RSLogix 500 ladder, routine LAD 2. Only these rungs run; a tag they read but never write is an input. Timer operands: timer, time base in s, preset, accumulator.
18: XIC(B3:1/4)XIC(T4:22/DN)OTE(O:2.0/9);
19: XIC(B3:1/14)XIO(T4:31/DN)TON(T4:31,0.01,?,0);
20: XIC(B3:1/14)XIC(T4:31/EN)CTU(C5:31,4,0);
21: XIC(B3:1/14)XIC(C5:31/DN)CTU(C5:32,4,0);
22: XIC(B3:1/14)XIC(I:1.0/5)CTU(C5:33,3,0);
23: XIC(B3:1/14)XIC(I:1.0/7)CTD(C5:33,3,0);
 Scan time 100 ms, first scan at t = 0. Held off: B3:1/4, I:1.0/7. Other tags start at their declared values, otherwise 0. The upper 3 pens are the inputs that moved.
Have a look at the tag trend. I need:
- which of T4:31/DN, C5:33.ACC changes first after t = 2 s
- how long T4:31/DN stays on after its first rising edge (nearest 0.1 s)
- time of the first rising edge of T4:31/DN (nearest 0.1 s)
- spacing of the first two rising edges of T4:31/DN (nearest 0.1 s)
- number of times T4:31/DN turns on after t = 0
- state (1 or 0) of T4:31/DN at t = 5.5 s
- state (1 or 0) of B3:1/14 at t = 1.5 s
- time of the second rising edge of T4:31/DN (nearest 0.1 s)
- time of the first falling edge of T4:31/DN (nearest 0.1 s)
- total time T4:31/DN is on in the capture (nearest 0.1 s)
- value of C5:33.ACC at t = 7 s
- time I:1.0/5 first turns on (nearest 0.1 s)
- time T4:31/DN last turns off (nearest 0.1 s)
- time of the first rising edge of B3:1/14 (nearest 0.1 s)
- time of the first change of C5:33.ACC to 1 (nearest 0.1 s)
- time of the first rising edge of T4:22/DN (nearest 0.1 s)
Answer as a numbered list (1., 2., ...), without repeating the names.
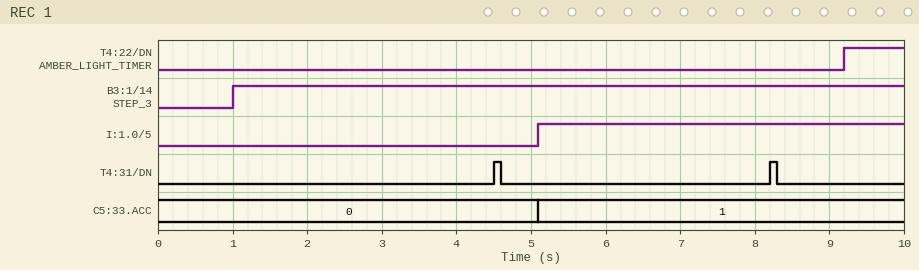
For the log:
1. T4:31/DN
2. 0.1 s
3. 4.5 s
4. 3.7 s
5. 2
6. 0
7. 1
8. 8.2 s
9. 4.6 s
10. 0.2 s
11. 1
12. 5.1 s
13. 8.3 s
14. 1.0 s
15. 5.1 s
16. 9.2 s
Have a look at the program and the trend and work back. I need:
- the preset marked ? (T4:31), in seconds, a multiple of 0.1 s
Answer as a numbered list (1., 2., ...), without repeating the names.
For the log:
1. 3.5 s
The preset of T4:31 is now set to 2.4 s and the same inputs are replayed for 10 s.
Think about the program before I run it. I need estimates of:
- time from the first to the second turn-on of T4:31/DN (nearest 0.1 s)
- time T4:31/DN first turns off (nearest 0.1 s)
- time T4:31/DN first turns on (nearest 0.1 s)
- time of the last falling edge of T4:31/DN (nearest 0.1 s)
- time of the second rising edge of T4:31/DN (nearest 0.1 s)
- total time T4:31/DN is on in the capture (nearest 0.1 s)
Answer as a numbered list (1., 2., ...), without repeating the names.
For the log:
1. 2.6 s
2. 3.5 s
3. 3.4 s
4. 8.7 s
5. 6.0 s
6. 0.3 s
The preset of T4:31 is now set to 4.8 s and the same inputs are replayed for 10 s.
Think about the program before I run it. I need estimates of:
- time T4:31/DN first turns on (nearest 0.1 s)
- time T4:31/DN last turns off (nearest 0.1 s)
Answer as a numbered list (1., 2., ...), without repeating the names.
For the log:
1. 5.8 s
2. 5.9 s
